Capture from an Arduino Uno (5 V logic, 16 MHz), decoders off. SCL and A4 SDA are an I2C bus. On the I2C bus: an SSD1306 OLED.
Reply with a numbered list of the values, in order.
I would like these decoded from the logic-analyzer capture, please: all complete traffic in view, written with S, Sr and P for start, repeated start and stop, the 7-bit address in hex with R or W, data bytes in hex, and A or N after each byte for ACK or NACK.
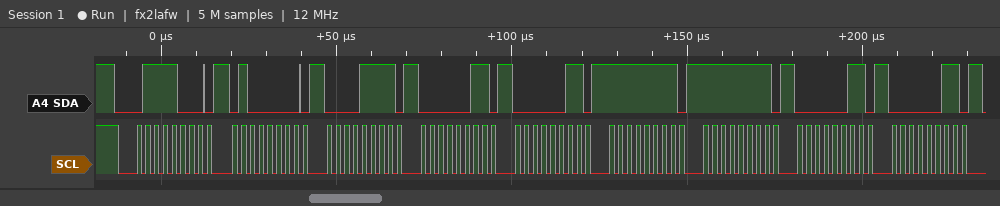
1. S 3CW A 40 A 0F A 03 A 03 A FF A FF A 03 A 03 A
